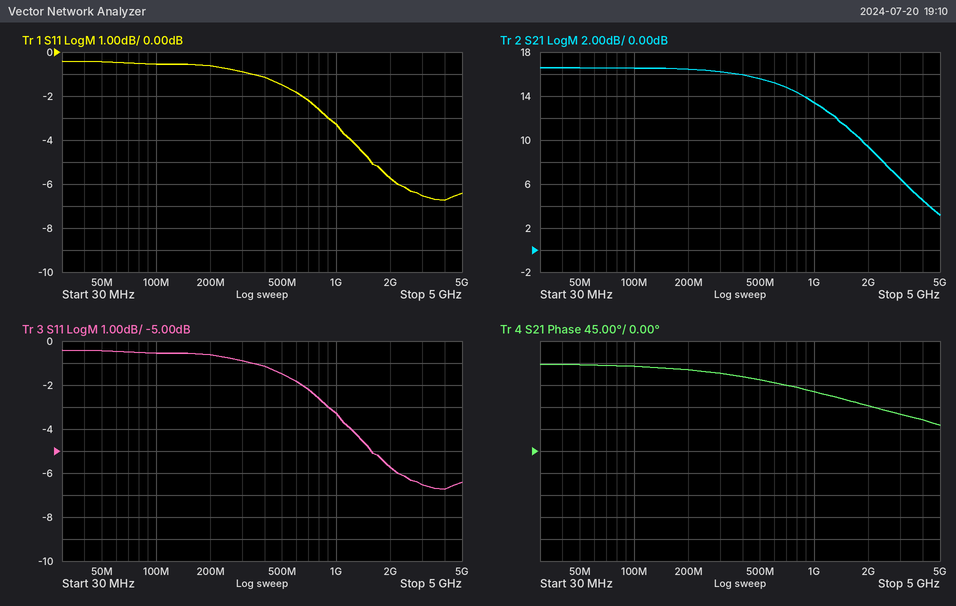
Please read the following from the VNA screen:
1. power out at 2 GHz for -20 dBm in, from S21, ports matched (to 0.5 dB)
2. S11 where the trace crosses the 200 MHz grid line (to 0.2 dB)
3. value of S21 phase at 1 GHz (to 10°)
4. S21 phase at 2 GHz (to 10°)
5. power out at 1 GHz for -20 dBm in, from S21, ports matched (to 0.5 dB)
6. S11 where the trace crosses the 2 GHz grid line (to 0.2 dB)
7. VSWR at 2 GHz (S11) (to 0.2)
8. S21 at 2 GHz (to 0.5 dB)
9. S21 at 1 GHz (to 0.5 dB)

-10.5 dBm
-0.6 dB
120°
90°
-6.5 dBm
-5.8 dB
3.2
9.5 dB
13.5 dB
